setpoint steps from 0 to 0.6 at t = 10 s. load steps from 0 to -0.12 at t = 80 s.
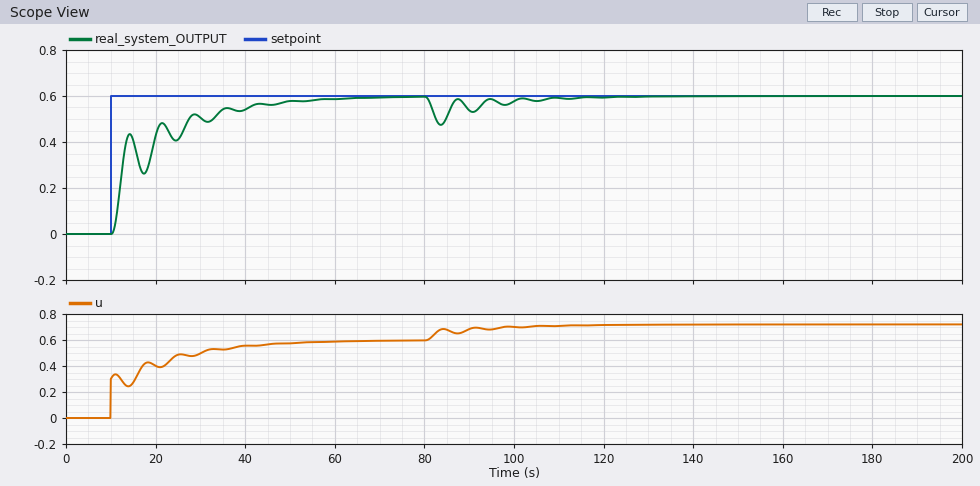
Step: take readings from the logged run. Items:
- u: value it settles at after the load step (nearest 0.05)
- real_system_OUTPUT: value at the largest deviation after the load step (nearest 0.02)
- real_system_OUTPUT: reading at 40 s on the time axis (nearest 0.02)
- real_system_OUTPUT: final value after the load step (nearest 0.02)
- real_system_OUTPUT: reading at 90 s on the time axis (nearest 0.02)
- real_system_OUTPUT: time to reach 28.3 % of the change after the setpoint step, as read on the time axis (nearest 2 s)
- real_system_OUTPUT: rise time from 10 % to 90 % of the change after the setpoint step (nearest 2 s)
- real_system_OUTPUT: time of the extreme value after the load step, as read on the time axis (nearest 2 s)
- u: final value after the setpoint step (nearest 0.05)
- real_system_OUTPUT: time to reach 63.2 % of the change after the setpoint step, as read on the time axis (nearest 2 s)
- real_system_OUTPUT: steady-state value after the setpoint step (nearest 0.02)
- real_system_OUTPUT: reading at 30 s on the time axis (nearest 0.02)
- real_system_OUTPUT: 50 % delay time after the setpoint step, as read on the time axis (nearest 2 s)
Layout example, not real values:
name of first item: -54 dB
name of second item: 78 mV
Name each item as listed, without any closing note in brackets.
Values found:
u: value it settles at after the load step: 0.70
real_system_OUTPUT: value at the largest deviation after the load step: 0.48
real_system_OUTPUT: reading at 40 s on the time axis: 0.54
real_system_OUTPUT: final value after the load step: 0.60
real_system_OUTPUT: reading at 90 s on the time axis: 0.54
real_system_OUTPUT: time to reach 28.3 % of the change after the setpoint step, as read on the time axis: 12 s
real_system_OUTPUT: rise time from 10 % to 90 % of the change after the setpoint step: 24 s
real_system_OUTPUT: time of the extreme value after the load step, as read on the time axis: 84 s
u: final value after the setpoint step: 0.60
real_system_OUTPUT: time to reach 63.2 % of the change after the setpoint step, as read on the time axis: 14 s
real_system_OUTPUT: steady-state value after the setpoint step: 0.60
real_system_OUTPUT: reading at 30 s on the time axis: 0.50
real_system_OUTPUT: 50 % delay time after the setpoint step, as read on the time axis: 12 s
